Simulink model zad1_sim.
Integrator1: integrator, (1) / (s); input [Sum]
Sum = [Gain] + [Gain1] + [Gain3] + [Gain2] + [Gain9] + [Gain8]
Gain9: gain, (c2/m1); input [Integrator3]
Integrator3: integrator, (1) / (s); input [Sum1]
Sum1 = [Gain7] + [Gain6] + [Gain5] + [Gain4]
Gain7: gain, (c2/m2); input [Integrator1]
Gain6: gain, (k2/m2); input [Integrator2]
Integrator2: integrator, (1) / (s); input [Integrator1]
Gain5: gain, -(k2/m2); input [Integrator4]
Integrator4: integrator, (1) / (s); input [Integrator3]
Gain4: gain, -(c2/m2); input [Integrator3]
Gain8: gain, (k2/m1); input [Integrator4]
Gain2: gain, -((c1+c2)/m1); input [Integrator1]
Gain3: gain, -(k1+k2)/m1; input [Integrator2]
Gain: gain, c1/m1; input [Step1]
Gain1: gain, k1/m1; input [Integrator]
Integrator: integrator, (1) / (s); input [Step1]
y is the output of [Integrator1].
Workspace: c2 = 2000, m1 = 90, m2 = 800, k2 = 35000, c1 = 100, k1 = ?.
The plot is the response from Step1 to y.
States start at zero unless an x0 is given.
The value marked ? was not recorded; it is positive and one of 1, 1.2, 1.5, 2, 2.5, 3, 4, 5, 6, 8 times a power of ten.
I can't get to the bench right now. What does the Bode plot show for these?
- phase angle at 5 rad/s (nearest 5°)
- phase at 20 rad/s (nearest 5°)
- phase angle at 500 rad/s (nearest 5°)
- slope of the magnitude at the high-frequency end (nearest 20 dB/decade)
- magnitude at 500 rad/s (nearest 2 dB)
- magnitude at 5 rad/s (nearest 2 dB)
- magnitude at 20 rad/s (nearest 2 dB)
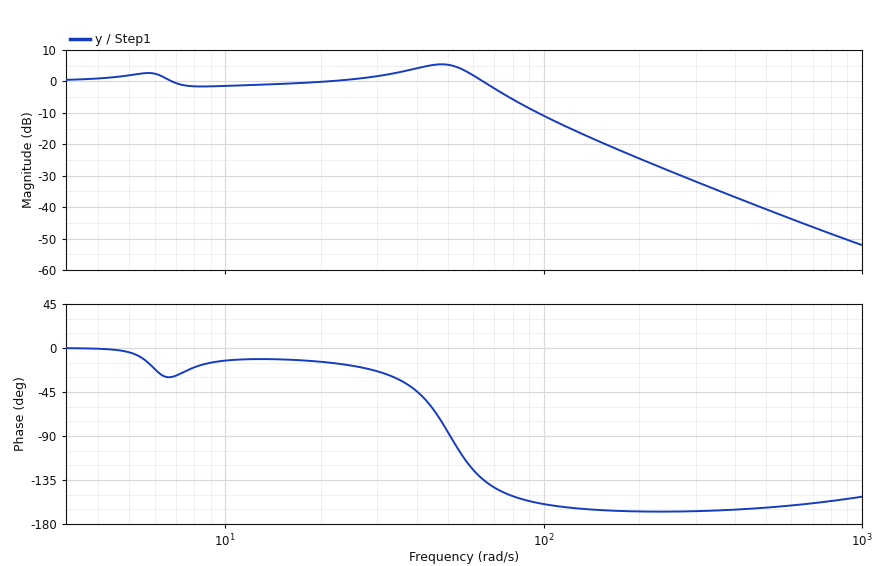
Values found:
-5°
-15°
-165°
-40 dB/decade
-40 dB
2 dB
0 dB
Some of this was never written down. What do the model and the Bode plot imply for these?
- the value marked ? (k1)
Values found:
200000
